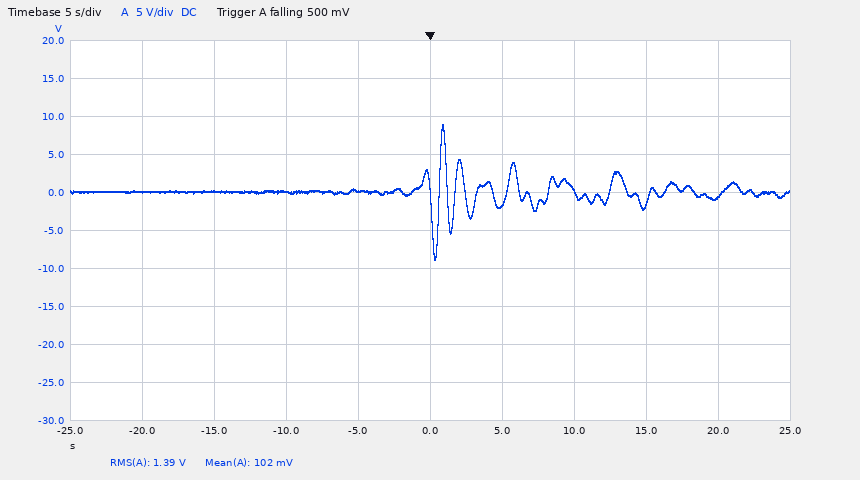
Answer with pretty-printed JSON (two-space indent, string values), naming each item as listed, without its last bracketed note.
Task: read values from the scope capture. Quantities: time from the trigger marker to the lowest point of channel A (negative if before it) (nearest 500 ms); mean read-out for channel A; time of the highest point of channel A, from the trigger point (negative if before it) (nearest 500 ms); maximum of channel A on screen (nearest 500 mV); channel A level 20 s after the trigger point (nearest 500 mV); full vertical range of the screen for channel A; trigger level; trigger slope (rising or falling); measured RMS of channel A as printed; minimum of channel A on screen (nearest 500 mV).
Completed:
{
  "time from the trigger marker to the lowest point of channel A (negative if before it)": "+500 ms",
  "mean read-out for channel A": "102 mV",
  "time of the highest point of channel A, from the trigger point (negative if before it)": "+1.0 s",
  "maximum of channel A on screen": "9.0 V",
  "channel A level 20 s after the trigger point": "-500 mV",
  "full vertical range of the screen for channel A": "50 V",
  "trigger level": "500 mV",
  "trigger slope": "falling",
  "measured RMS of channel A as printed": "1.39 V",
  "minimum of channel A on screen": "-9.0 V"
}
